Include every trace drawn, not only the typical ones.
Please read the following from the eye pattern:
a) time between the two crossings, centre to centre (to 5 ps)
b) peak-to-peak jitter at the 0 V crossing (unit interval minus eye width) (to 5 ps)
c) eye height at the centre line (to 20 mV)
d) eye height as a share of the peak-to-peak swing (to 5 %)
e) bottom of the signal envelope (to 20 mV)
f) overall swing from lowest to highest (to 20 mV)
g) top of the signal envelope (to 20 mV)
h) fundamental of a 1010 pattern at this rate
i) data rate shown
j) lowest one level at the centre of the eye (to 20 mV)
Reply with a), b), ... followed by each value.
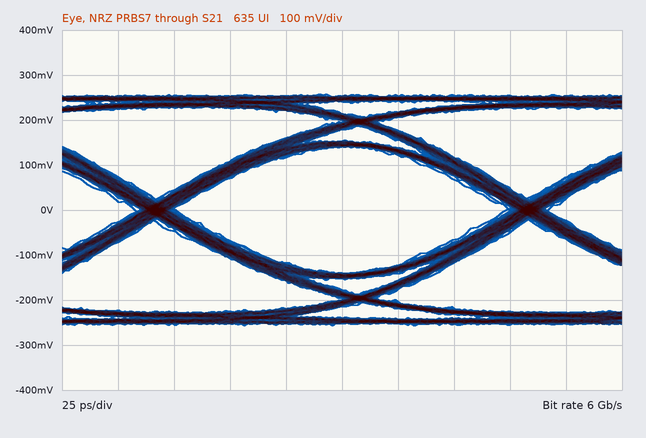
a) 165 ps
b) 20 ps
c) 280 mV
d) 55 %
e) -260 mV
f) 520 mV
g) 260 mV
h) 3 GHz
i) 6 Gb/s
j) 140 mV
